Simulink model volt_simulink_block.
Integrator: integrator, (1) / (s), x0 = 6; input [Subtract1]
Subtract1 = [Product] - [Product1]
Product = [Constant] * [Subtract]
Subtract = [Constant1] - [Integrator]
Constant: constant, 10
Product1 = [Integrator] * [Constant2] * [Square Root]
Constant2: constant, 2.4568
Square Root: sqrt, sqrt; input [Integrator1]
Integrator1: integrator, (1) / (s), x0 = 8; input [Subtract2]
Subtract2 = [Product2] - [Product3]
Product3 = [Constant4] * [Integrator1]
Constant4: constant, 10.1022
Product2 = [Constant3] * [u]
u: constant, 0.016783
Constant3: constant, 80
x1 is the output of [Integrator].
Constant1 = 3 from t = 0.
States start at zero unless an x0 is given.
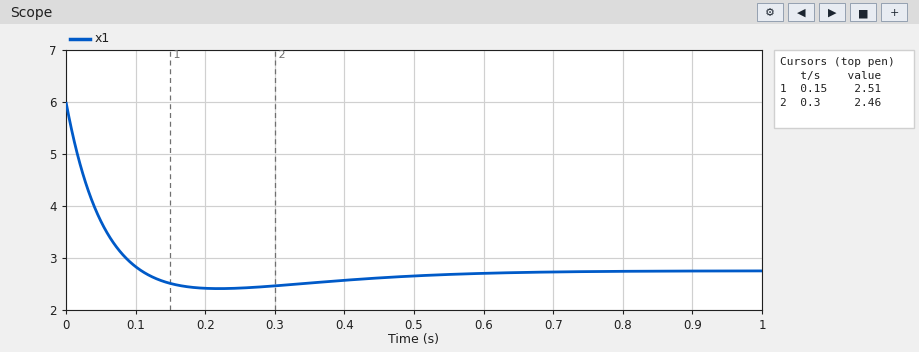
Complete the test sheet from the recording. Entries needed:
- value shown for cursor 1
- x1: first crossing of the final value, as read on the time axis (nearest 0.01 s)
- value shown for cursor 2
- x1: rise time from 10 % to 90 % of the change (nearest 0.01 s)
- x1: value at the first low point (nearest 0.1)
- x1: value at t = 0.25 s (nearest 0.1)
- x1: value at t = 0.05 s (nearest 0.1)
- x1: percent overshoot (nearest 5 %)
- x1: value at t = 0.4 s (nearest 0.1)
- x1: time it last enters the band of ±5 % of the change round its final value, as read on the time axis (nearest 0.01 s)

2.51
0.11 s
2.46
0.08 s
2.4
2.4
3.7
10 %
2.6
0.42 s
